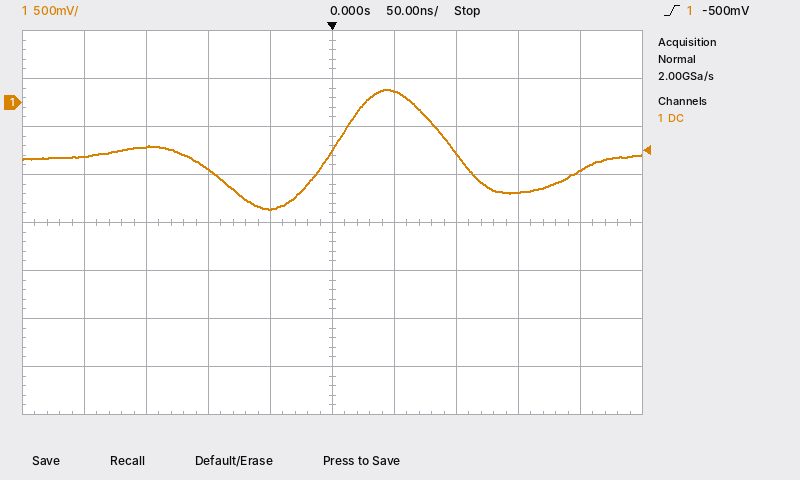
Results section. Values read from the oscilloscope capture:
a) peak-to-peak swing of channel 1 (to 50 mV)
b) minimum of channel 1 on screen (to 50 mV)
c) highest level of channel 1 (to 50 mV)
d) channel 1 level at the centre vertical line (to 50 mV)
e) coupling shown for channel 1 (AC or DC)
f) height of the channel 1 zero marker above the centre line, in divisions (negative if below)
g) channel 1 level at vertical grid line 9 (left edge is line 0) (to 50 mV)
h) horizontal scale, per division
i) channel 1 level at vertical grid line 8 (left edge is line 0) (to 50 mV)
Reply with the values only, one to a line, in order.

1.25 V
-1.10 V
150 mV
-500 mV
DC
+2.5 div
-700 mV
50 ns
-950 mV
